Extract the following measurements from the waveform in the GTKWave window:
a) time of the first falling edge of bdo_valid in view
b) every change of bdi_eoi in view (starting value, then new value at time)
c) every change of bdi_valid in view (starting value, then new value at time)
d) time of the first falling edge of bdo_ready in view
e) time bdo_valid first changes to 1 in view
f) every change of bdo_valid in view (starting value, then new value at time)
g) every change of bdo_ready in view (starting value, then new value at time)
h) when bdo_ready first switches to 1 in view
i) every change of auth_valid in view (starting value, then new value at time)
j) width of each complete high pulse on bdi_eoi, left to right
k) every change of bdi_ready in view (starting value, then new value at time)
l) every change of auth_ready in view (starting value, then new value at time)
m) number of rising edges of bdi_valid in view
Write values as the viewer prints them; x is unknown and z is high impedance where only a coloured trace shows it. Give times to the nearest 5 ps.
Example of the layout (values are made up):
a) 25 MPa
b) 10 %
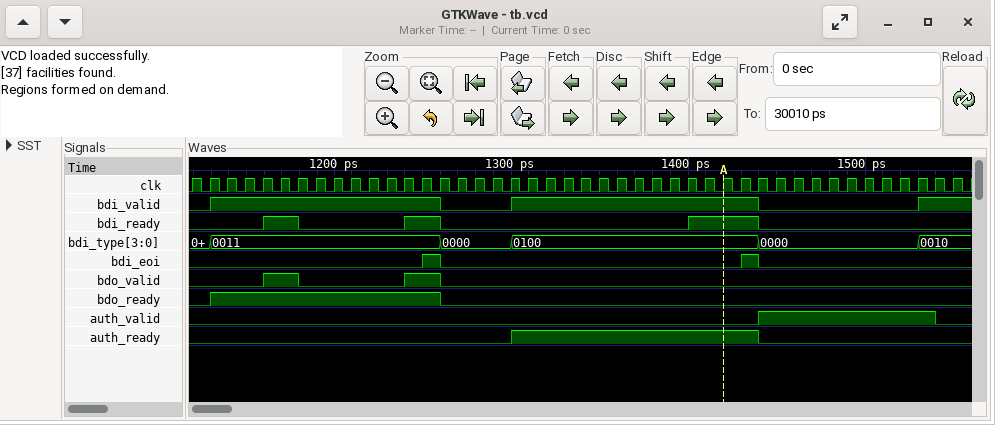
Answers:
a) 1180 ps
b) 0, 1 at 1250 ps, 0 at 1260 ps, 1 at 1430 ps, 0 at 1440 ps
c) 0, 1 at 1130 ps, 0 at 1260 ps, 1 at 1300 ps, 0 at 1440 ps, 1 at 1530 ps
d) 1260 ps
e) 1160 ps
f) 0, 1 at 1160 ps, 0 at 1180 ps, 1 at 1240 ps, 0 at 1260 ps
g) 0, 1 at 1130 ps, 0 at 1260 ps
h) 1130 ps
i) 0, 1 at 1440 ps, 0 at 1540 ps
j) 10 ps, 10 ps
k) 0, 1 at 1160 ps, 0 at 1180 ps, 1 at 1240 ps, 0 at 1260 ps, 1 at 1400 ps, 0 at 1440 ps
l) 0, 1 at 1300 ps, 0 at 1440 ps
m) 3
